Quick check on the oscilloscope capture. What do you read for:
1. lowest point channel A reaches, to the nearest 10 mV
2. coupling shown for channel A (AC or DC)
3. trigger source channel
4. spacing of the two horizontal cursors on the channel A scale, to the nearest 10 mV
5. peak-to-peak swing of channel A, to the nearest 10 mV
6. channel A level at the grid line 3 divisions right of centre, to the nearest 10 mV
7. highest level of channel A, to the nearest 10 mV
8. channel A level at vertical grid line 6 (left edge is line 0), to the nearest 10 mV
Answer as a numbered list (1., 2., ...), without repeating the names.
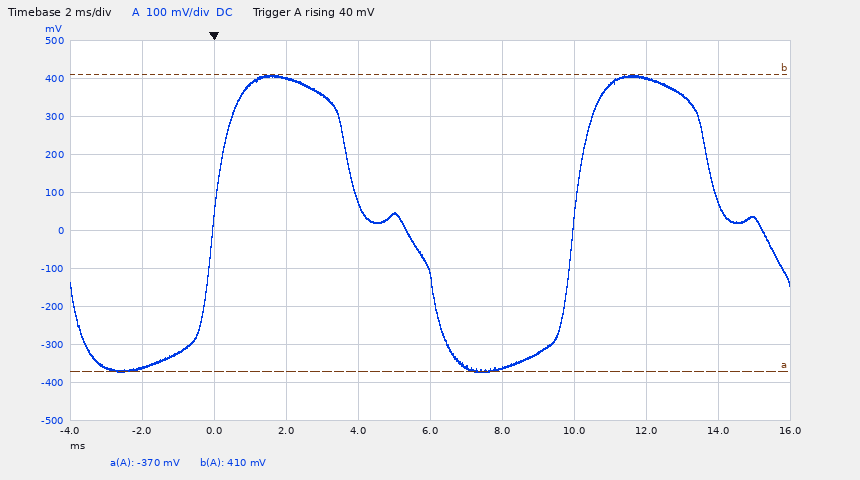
1. -370 mV
2. DC
3. channel A
4. 780 mV
5. 780 mV
6. 400 mV
7. 410 mV
8. -360 mV
